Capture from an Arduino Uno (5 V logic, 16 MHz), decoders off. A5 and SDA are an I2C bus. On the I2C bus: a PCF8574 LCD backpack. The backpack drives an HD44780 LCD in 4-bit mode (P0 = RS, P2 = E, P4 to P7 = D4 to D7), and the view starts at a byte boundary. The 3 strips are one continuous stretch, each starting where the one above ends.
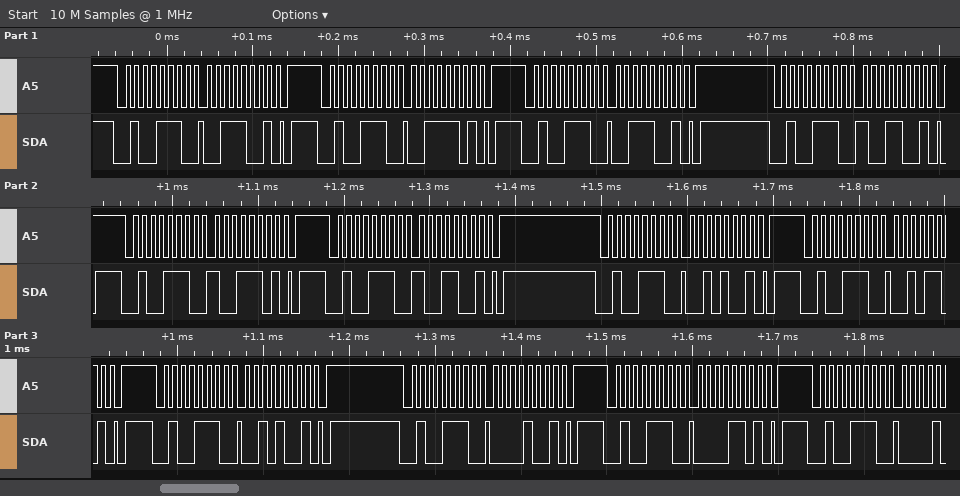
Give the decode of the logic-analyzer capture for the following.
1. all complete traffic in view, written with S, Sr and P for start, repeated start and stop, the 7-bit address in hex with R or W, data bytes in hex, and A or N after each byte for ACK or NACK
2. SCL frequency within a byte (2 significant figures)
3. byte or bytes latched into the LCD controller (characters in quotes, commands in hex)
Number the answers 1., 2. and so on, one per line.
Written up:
1. S 27W A 39 A P S 27W A 3D A P S 27W A 39 A P S 27W A 99 A P S 27W A 9D A P S 27W A 99 A P S 27W A 29 A P S 27W A 2D A P S 27W A 29 A P S 27W A 09 A P S 27W A 0D A P S 27W A
2. 100 kHz
3. '9'
